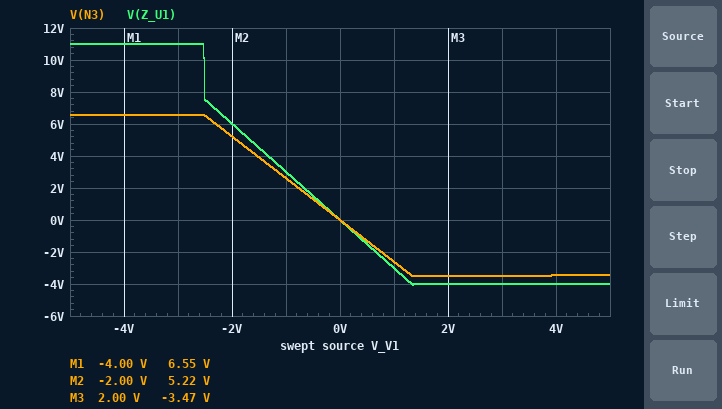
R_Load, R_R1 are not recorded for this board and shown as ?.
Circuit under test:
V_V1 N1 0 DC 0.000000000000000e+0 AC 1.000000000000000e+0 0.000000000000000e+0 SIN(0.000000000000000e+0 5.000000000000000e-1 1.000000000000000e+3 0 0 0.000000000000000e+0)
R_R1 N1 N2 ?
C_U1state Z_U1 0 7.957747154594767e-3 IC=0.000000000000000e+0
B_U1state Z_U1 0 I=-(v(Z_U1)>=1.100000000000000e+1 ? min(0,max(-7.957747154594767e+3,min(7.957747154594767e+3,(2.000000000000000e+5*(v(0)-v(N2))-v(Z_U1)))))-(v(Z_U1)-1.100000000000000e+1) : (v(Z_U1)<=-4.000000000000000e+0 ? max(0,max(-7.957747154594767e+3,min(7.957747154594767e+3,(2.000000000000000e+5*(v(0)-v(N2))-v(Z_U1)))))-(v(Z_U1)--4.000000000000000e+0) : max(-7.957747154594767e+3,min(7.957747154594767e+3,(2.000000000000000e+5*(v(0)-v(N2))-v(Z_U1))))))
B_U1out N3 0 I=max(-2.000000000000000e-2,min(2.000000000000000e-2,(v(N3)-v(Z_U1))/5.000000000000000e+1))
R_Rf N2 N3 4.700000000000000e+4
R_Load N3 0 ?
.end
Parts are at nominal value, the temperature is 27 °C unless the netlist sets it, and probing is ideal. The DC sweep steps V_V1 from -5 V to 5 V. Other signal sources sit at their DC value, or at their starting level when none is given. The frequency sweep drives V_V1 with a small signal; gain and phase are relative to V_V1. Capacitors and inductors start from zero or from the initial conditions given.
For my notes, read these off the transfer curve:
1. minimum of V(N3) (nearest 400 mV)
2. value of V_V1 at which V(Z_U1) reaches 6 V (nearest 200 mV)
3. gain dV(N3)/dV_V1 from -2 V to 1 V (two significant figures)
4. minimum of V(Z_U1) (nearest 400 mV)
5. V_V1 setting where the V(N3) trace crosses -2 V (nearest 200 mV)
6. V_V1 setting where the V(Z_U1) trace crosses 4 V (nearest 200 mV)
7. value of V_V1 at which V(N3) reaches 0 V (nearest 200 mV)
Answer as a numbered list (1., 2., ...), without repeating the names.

1. -3.6 V
2. -2.0 V
3. -2.6 V/V
4. -4.0 V
5. 800 mV
6. -1.4 V
7. 0 V
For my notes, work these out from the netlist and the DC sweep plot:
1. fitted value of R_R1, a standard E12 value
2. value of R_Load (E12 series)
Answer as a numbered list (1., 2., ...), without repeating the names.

1. 18 kΩ
2. 330 Ω
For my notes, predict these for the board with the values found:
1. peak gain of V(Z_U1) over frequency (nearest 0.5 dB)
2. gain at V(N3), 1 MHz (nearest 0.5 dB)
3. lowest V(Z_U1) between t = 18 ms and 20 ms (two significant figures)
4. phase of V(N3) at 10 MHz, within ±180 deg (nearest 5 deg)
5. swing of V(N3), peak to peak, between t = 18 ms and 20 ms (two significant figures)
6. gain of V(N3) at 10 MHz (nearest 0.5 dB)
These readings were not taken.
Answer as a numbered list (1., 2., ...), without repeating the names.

1. 9.5 dB
2. 5.0 dB
3. -1.5 V
4. 95 deg
5. 2.6 V
6. -12.0 dB
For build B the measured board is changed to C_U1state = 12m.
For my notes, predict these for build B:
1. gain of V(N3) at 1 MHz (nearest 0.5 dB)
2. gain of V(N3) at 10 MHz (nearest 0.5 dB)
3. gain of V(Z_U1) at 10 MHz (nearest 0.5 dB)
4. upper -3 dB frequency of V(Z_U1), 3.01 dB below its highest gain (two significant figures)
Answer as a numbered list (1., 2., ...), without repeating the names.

1. 3.0 dB
2. -15.5 dB
3. -14.5 dB
4. 640 kHz
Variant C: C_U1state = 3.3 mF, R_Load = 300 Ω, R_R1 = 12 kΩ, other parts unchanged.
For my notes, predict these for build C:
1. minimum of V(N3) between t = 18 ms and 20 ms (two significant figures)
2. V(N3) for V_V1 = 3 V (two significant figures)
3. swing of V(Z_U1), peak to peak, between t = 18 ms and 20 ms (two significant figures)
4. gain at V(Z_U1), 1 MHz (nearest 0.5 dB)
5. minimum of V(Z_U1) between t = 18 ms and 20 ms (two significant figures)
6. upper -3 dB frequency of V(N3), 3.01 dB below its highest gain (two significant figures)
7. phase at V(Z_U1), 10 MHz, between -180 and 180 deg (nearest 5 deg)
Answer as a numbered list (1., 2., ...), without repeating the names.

1. -2.0 V
2. -3.4 V
3. 4.6 V
4. 12.0 dB
5. -2.3 V
6. 1.7 MHz
7. 100 deg
